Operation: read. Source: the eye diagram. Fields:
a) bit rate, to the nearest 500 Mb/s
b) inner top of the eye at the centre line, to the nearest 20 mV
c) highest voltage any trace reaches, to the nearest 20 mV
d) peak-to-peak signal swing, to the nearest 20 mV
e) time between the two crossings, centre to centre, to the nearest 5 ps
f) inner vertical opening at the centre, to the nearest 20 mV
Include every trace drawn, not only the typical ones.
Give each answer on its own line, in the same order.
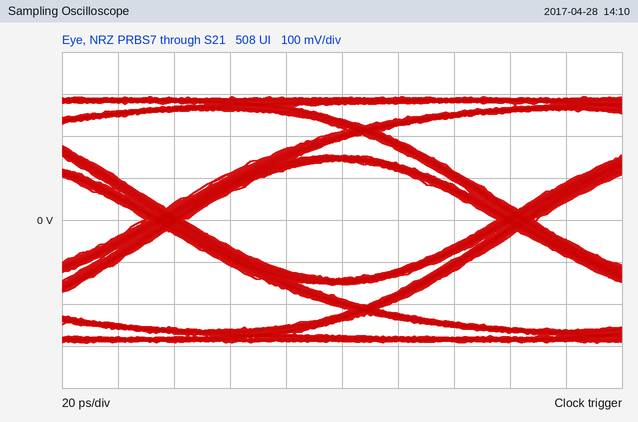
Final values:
8.0 Gb/s
140 mV
300 mV
580 mV
125 ps
280 mV
